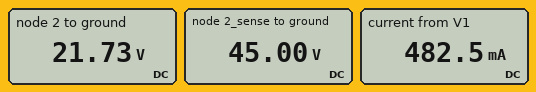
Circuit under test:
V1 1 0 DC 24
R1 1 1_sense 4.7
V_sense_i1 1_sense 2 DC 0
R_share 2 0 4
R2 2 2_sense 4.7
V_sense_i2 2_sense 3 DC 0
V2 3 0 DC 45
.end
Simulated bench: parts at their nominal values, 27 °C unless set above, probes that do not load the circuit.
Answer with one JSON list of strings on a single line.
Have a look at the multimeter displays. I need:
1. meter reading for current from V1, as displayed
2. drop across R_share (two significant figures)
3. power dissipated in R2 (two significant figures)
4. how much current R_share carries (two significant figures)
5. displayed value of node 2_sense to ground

["482.5 mA", "22 V", "120 W", "5.4 A", "45.00 V"]
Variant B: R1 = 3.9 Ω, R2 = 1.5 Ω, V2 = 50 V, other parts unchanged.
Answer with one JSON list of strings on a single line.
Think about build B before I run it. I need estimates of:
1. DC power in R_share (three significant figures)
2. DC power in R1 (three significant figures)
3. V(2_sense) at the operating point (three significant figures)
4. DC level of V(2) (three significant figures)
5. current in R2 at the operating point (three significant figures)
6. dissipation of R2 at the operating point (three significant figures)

["283 W", "23.9 W", "50.0 V", "33.7 V", "10.9 A", "178 W"]
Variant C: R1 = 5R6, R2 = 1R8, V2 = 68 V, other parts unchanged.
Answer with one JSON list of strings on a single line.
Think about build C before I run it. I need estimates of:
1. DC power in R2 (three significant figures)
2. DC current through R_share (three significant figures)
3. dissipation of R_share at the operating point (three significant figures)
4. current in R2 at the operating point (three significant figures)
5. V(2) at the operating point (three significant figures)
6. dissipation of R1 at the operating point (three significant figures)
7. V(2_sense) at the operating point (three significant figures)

["354 W", "10.7 A", "457 W", "14.0 A", "42.7 V", "62.7 W", "68.0 V"]
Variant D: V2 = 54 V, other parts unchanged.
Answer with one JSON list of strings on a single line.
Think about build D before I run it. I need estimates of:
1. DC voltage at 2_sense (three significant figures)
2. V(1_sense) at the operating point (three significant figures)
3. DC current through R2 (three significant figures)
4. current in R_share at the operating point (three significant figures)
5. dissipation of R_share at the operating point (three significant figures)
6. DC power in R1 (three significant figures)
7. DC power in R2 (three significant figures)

["54.0 V", "24.6 V", "6.26 A", "6.14 A", "151 W", "68.4 mW", "184 W"]
